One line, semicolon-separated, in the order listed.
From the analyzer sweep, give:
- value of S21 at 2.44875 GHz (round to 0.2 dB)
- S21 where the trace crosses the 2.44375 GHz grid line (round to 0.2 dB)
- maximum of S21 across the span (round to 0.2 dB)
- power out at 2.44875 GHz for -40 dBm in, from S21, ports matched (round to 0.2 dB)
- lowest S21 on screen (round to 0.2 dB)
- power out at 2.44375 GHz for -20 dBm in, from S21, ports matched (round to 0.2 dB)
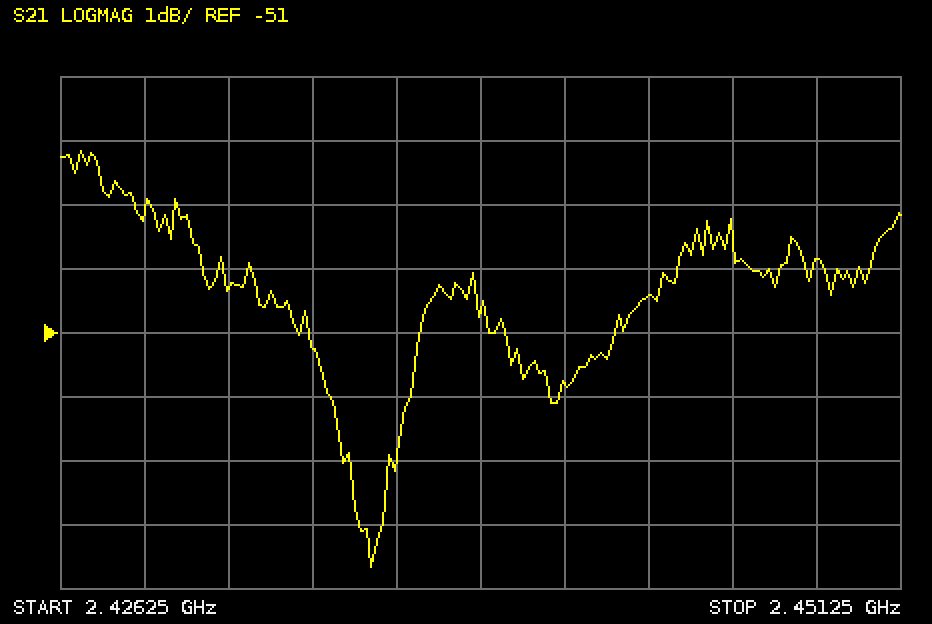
-49.8 dB; -50.4 dB; -48.2 dB; -89.8 dBm; -54.6 dB; -70.4 dBm
